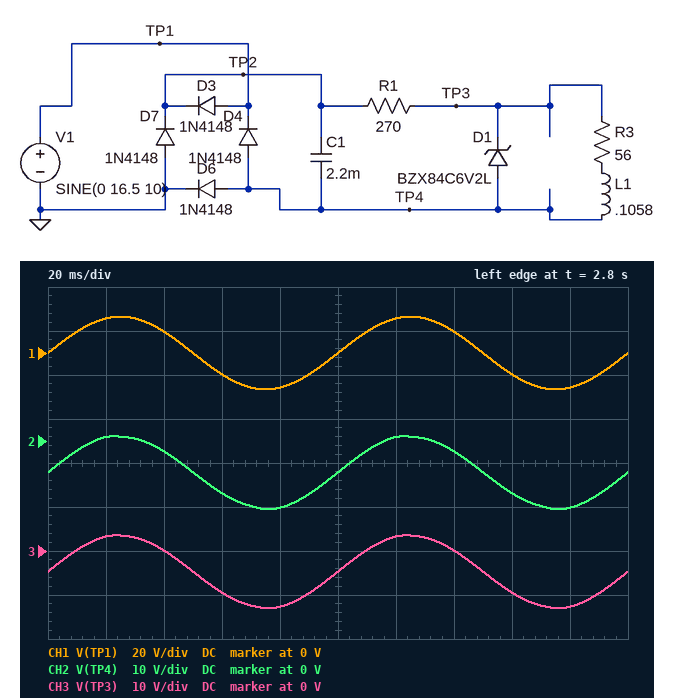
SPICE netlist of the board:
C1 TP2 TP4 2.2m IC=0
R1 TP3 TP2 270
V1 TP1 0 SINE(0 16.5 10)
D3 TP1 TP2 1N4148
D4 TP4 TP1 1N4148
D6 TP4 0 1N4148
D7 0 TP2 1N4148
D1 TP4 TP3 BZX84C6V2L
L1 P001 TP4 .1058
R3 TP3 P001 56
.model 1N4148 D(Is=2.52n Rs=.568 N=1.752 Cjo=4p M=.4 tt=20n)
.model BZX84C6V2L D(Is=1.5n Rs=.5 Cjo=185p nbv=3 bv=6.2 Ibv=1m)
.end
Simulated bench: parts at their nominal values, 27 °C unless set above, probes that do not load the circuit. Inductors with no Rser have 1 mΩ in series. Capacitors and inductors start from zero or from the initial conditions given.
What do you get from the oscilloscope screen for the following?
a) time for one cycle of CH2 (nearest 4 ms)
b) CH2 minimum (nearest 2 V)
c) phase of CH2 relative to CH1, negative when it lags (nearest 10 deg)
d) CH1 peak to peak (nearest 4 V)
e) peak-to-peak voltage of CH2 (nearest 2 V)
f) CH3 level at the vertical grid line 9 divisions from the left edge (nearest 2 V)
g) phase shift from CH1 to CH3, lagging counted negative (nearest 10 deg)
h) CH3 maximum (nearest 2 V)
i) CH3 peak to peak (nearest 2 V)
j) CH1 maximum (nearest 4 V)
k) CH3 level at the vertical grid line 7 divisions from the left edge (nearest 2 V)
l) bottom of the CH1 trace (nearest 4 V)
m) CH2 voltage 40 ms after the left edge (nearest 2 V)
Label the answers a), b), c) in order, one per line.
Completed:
a) 100 ms
b) -16 V
c) 0 deg
d) 32 V
e) 16 V
f) -12 V
g) 0 deg
h) 4 V
i) 16 V
j) 16 V
k) 0 V
l) -16 V
m) -2 V
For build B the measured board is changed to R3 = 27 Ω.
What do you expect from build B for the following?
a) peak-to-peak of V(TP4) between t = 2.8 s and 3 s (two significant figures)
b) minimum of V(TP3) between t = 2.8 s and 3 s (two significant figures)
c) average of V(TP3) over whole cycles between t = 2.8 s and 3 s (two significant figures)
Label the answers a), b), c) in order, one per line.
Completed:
a) 17 V
b) -14 V
c) -5.8 V
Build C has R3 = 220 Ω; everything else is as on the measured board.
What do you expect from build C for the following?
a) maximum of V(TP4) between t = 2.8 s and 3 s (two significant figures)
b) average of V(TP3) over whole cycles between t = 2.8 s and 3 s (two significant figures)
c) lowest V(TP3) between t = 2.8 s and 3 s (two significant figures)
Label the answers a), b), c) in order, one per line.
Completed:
a) 1.0 V
b) -970 mV
c) -9.3 V
